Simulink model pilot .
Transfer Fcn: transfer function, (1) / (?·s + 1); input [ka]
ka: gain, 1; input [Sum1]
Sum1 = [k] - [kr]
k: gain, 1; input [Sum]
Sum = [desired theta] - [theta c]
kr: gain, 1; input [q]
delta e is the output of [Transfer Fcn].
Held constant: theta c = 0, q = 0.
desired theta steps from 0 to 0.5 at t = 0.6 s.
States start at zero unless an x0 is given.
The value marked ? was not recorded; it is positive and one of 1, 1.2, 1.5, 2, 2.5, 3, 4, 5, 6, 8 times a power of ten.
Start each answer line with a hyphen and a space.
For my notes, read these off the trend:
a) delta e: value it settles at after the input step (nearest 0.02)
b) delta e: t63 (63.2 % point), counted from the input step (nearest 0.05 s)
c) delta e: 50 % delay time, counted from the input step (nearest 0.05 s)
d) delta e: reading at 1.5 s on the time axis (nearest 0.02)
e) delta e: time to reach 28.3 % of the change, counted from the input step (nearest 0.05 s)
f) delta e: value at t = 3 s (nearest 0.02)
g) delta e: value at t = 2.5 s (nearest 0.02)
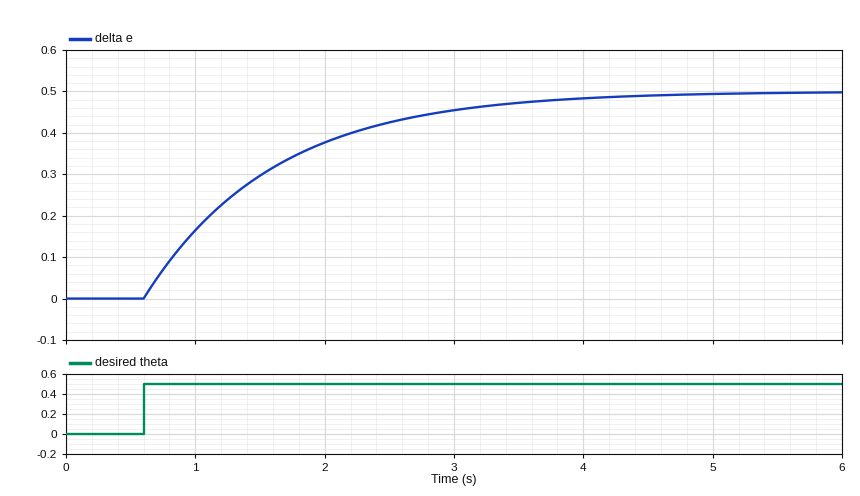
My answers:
- 0.50
- 1.00 s
- 0.70 s
- 0.30
- 0.35 s
- 0.46
- 0.42
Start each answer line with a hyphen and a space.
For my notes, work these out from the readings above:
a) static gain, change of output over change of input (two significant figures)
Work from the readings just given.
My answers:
- 1.0
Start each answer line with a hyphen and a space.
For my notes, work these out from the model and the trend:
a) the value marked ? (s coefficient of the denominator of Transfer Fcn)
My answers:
- 1
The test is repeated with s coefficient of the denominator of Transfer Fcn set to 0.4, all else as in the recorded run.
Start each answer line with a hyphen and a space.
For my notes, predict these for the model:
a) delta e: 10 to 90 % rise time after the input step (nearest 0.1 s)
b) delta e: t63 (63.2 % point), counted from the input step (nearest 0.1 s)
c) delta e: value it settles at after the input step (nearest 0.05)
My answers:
- 0.9 s
- 0.4 s
- 0.50
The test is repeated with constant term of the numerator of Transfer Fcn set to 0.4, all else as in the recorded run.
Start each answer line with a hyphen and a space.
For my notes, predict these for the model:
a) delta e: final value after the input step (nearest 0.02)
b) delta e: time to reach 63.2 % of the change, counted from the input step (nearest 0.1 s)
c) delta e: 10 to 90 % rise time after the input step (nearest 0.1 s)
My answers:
- 0.20
- 1.0 s
- 2.2 s
